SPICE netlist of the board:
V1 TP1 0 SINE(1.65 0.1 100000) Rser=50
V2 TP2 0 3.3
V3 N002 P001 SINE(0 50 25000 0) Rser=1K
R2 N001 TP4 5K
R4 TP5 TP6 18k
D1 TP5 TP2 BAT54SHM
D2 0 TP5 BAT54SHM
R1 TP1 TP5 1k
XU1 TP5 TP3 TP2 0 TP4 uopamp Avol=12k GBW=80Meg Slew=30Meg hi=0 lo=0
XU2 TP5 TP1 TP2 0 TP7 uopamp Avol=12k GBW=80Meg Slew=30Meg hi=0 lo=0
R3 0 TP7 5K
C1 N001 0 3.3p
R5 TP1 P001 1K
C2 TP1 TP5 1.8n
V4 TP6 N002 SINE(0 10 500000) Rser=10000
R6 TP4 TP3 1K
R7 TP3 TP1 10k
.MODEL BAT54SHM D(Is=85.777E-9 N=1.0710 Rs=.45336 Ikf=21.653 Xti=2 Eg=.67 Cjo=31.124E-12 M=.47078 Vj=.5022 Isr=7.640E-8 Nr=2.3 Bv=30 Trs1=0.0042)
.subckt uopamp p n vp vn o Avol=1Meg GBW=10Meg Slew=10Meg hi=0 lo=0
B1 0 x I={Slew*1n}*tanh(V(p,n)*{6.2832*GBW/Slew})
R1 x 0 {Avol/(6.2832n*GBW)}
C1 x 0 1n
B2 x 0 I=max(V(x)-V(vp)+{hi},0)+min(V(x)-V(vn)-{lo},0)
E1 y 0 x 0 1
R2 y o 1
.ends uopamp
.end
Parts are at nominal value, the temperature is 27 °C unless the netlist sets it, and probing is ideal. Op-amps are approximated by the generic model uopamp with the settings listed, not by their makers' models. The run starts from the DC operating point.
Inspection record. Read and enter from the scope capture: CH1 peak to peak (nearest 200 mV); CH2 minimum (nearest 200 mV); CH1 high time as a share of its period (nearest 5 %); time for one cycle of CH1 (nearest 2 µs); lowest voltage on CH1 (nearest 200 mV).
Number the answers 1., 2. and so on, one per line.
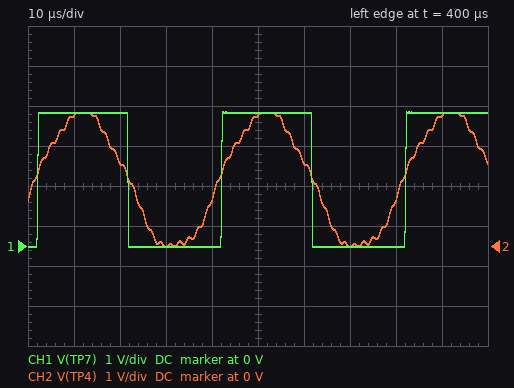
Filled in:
1. 3.4 V
2. 0 V
3. 50 %
4. 40 µs
5. 0 V
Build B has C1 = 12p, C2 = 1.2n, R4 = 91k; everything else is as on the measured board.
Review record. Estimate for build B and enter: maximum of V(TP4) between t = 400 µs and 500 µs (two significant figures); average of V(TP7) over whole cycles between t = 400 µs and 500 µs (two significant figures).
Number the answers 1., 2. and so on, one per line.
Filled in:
1. 2.3 V
2. 1.7 V
